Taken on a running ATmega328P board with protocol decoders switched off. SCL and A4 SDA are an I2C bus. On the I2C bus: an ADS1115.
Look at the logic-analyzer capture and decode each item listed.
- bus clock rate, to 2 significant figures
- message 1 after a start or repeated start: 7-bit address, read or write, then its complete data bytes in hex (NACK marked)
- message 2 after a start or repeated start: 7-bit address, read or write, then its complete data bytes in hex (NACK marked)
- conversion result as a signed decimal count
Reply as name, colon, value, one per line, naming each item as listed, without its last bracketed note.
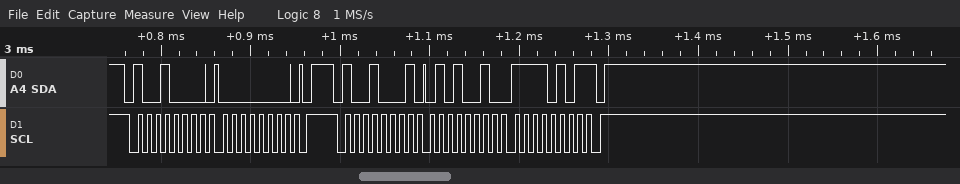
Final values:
bus clock rate, to 2 significant figures: 100 kHz
message 1 after a start or repeated start: 7-bit address, read or write, then its complete data bytes in hex: 0x48 write: 00
message 2 after a start or repeated start: 7-bit address, read or write, then its complete data bytes in hex: 0x48 read: 52 F5 NACK
conversion result as a signed decimal count: 21237
